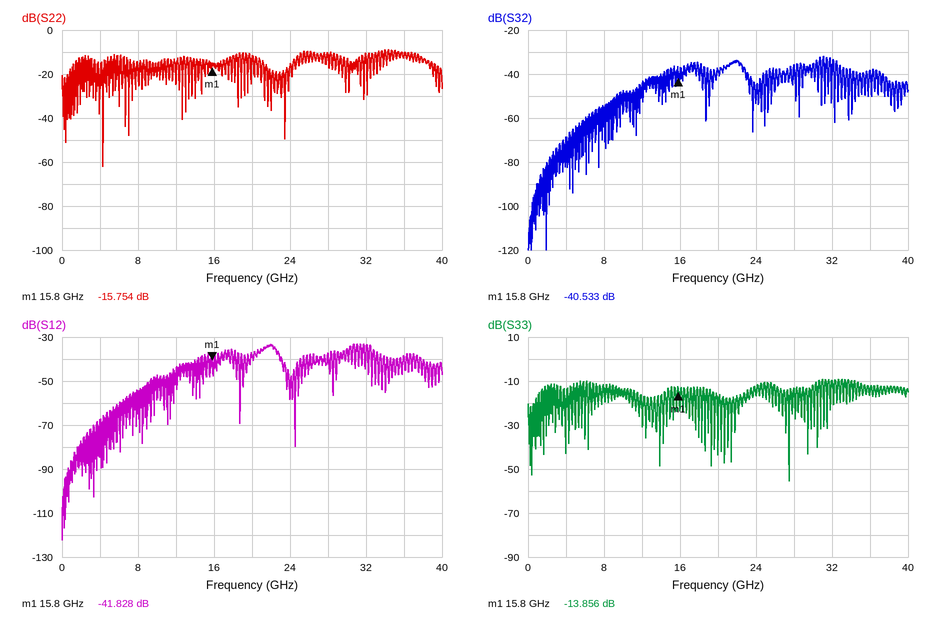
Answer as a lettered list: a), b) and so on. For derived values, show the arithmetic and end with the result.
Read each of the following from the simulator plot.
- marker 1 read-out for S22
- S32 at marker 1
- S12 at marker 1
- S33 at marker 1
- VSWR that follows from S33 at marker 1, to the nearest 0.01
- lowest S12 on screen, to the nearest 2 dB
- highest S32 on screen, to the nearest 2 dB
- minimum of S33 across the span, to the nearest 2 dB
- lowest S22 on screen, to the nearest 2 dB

a) -15.754 dB
b) -40.533 dB
c) -41.828 dB
d) -13.856 dB
e) (1 + 0.2029)/(1 − 0.2029) ≈ 1.51
f) -122 dB
g) -32 dB
h) -56 dB
i) -62 dB
